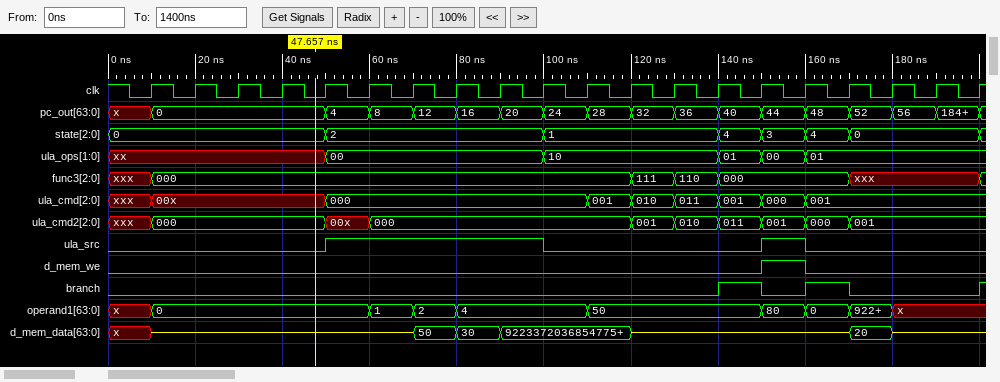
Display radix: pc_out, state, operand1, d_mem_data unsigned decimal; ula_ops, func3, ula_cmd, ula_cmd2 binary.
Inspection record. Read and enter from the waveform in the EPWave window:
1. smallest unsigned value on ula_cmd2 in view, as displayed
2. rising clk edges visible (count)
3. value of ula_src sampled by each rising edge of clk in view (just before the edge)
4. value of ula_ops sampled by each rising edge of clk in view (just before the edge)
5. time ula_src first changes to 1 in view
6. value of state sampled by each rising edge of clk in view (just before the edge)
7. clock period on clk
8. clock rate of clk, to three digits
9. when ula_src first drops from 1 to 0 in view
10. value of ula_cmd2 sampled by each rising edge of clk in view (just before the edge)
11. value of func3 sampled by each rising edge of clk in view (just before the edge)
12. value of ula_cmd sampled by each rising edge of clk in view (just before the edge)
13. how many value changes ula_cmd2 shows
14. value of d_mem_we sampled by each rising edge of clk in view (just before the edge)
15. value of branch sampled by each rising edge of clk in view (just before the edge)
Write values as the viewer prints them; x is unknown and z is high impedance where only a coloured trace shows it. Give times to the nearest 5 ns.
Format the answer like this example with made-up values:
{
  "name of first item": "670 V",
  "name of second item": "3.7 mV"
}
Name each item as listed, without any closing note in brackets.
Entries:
{
  "smallest unsigned value on ula_cmd2 in view, as displayed": "000",
  "rising clk edges visible": "20",
  "value of ula_src sampled by each rising edge of clk in view": "0 0 0 0 0 1 1 1 1 1 0 0 0 0 0 1 0 0 0 0",
  "value of ula_ops sampled by each rising edge of clk in view": "xx, xx, xx, xx, xx, 00, 00, 00, 00, 00, 10, 10, 10, 10, 01, 00, 01, 01, 01, 01",
  "time ula_src first changes to 1 in view": "50 ns",
  "value of state sampled by each rising edge of clk in view": "0, 0, 0, 0, 0, 2, 2, 2, 2, 2, 1, 1, 1, 1, 4, 3, 4, 0, 0, 0",
  "clock period on clk": "10 ns",
  "clock rate of clk, to three digits": "100 MHz",
  "when ula_src first drops from 1 to 0 in view": "100 ns",
  "value of ula_cmd2 sampled by each rising edge of clk in view": "xxx, 000, 000, 000, 000, 00x, 000, 000, 000, 000, 000, 000, 001, 010, 011, 001, 000, 001, 001, 001",
  "value of func3 sampled by each rising edge of clk in view": "xxx, 000, 000, 000, 000, 000, 000, 000, 000, 000, 000, 000, 111, 110, 000, 000, 000, xxx, xxx, xxx",
  "value of ula_cmd sampled by each rising edge of clk in view": "xxx, 00x, 00x, 00x, 00x, 000, 000, 000, 000, 000, 000, 001, 010, 011, 001, 000, 001, 001, 001, 001",
  "how many value changes ula_cmd2 shows": "9",
  "value of d_mem_we sampled by each rising edge of clk in view": "0 0 0 0 0 0 0 0 0 0 0 0 0 0 0 1 0 0 0 0",
  "value of branch sampled by each rising edge of clk in view": "0 0 0 0 0 0 0 0 0 0 0 0 0 0 1 0 1 0 0 0"
}
